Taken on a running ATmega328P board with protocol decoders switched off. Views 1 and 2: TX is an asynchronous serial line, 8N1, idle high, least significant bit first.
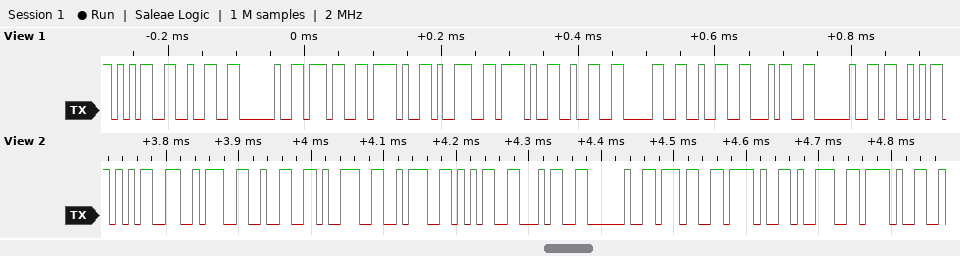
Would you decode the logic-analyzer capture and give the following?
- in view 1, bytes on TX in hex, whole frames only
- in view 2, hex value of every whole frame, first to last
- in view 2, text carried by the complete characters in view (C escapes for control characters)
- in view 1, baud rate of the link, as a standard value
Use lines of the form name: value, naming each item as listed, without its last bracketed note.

in view 1, bytes on TX in hex, whole frames only: 35 32 20 37 2F 39 2F 32 30 32 34 20 53
in view 2, hex value of every whole frame, first to last: 0x35 0x3A 0x32 0x39 0x3A 0x35 0x34 0x20 0x37 0x2F 0x39 0x2F
in view 2, text carried by the complete characters in view: "5:29:54 7/9/"
in view 1, baud rate of the link, as a standard value: 115200 baud
